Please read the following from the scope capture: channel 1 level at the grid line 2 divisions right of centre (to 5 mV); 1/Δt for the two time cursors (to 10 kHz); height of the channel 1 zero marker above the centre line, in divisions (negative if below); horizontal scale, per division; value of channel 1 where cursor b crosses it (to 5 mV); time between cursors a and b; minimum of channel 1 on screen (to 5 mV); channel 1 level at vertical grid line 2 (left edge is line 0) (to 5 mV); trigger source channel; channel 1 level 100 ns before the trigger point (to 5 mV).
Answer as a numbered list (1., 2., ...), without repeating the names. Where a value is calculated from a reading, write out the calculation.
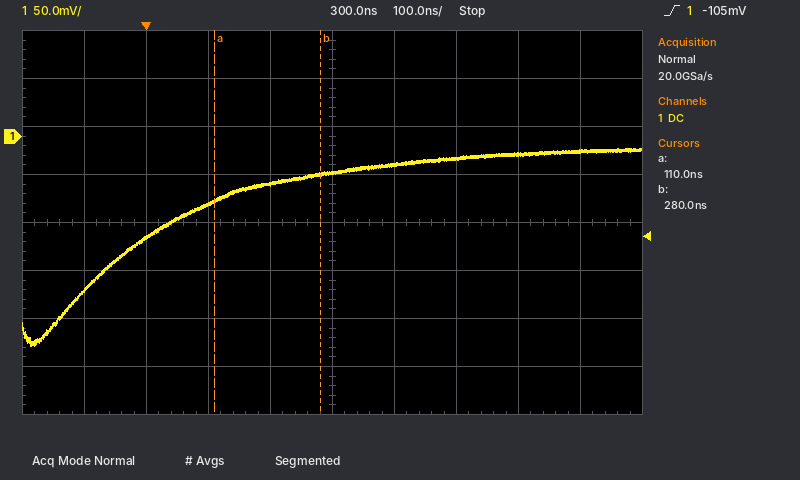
1. -25 mV
2. 1 / 170 ns ≈ 5.88 MHz
3. +1.8 div
4. 100 ns
5. -40 mV
6. 280 ns − (110 ns) = 170 ns
7. -220 mV
8. -105 mV
9. channel 1
10. -160 mV
